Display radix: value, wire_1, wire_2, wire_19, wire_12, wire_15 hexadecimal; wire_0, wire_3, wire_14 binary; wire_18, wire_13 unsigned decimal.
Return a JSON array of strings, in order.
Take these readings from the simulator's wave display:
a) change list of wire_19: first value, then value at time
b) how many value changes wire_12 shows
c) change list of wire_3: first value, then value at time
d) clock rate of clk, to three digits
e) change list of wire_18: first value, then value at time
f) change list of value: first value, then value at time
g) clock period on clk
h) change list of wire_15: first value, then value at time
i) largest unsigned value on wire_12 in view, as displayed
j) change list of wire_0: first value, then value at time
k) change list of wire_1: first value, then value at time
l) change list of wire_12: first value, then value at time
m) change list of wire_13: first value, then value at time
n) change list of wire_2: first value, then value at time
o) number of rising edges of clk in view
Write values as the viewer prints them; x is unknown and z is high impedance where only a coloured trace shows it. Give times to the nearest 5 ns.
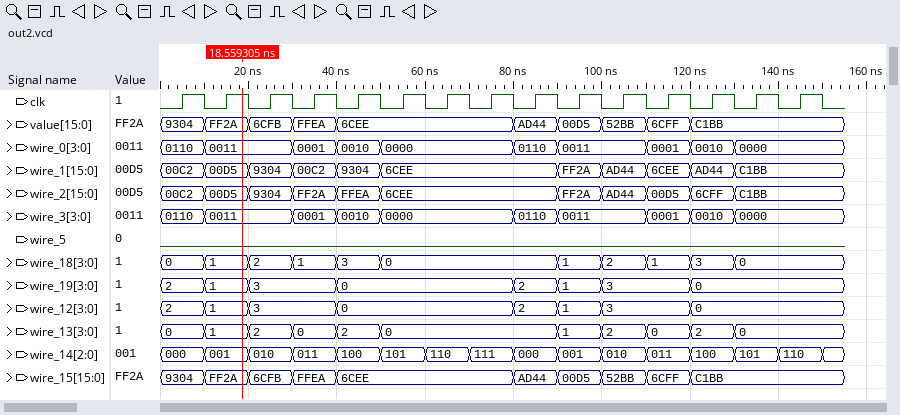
["2, 1 at 10 ns, 3 at 20 ns, 0 at 40 ns, 2 at 80 ns, 1 at 90 ns, 3 at 100 ns, 0 at 120 ns", "7", "0110, 0011 at 10 ns, 0001 at 30 ns, 0010 at 40 ns, 0000 at 50 ns, 0110 at 80 ns, 0011 at 90 ns, 0001 at 110 ns, 0010 at 120 ns, 0000 at 130 ns", "100 MHz", "0, 1 at 10 ns, 2 at 20 ns, 1 at 30 ns, 3 at 40 ns, 0 at 50 ns, 1 at 90 ns, 2 at 100 ns, 1 at 110 ns, 3 at 120 ns, 0 at 130 ns", "9304, FF2A at 10 ns, 6CFB at 20 ns, FFEA at 30 ns, 6CEE at 40 ns, AD44 at 80 ns, 00D5 at 90 ns, 52BB at 100 ns, 6CFF at 110 ns, C1BB at 120 ns", "10 ns", "9304, FF2A at 10 ns, 6CFB at 20 ns, FFEA at 30 ns, 6CEE at 40 ns, AD44 at 80 ns, 00D5 at 90 ns, 52BB at 100 ns, 6CFF at 110 ns, C1BB at 120 ns", "3", "0110, 0011 at 10 ns, 0001 at 30 ns, 0010 at 40 ns, 0000 at 50 ns, 0110 at 80 ns, 0011 at 90 ns, 0001 at 110 ns, 0010 at 120 ns, 0000 at 130 ns", "00C2, 00D5 at 10 ns, 9304 at 20 ns, 00C2 at 30 ns, 9304 at 40 ns, 6CEE at 50 ns, FF2A at 90 ns, AD44 at 100 ns, 6CEE at 110 ns, AD44 at 120 ns, C1BB at 130 ns", "2, 1 at 10 ns, 3 at 20 ns, 0 at 40 ns, 2 at 80 ns, 1 at 90 ns, 3 at 100 ns, 0 at 120 ns", "0, 1 at 10 ns, 2 at 20 ns, 0 at 30 ns, 2 at 40 ns, 0 at 50 ns, 1 at 90 ns, 2 at 100 ns, 0 at 110 ns, 2 at 120 ns, 0 at 130 ns", "00C2, 00D5 at 10 ns, 9304 at 20 ns, FF2A at 30 ns, FFEA at 40 ns, 6CEE at 50 ns, FF2A at 90 ns, AD44 at 100 ns, 00D5 at 110 ns, 6CFF at 120 ns, C1BB at 130 ns", "15"]
